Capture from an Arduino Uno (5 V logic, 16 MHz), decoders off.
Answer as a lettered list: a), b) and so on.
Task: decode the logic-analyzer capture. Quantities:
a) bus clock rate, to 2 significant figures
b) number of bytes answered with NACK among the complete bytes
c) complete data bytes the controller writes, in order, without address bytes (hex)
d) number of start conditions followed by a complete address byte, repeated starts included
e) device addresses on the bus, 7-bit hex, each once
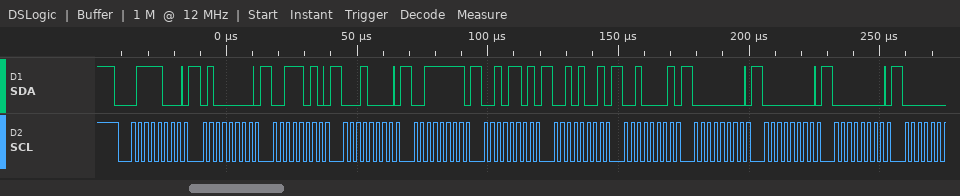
a) 400 kHz
b) 0
c) 40 3A 10 3F 2D 29 21 00 00 00
d) 1
e) 0x3C
